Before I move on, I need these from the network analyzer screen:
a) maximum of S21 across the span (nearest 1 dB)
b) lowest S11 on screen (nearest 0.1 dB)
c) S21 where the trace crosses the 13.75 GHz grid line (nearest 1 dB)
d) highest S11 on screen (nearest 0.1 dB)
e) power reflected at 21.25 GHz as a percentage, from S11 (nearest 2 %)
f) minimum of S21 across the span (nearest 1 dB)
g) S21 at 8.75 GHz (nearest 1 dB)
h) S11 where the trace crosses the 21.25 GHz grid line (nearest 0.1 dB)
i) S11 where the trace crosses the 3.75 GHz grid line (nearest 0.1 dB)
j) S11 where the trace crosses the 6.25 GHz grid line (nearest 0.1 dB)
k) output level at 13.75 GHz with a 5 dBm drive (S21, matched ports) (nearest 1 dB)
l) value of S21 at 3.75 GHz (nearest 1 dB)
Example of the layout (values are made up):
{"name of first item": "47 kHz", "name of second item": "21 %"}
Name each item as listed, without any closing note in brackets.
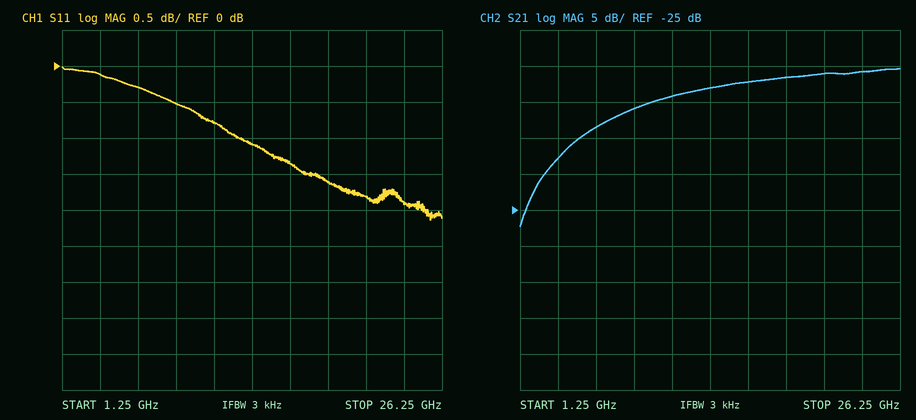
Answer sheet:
{"maximum of S21 across the span": "-5 dB", "lowest S11 on screen": "-2.1 dB", "S21 where the trace crosses the 13.75 GHz grid line": "-8 dB", "highest S11 on screen": "0.0 dB", "power reflected at 21.25 GHz as a percentage, from S11": "66 %", "minimum of S21 across the span": "-27 dB", "S21 at 8.75 GHz": "-11 dB", "S11 where the trace crosses the 21.25 GHz grid line": "-1.8 dB", "S11 where the trace crosses the 3.75 GHz grid line": "-0.1 dB", "S11 where the trace crosses the 6.25 GHz grid line": "-0.3 dB", "output level at 13.75 GHz with a 5 dBm drive (S21, matched ports)": "-3 dBm", "value of S21 at 3.75 GHz": "-18 dB"}
